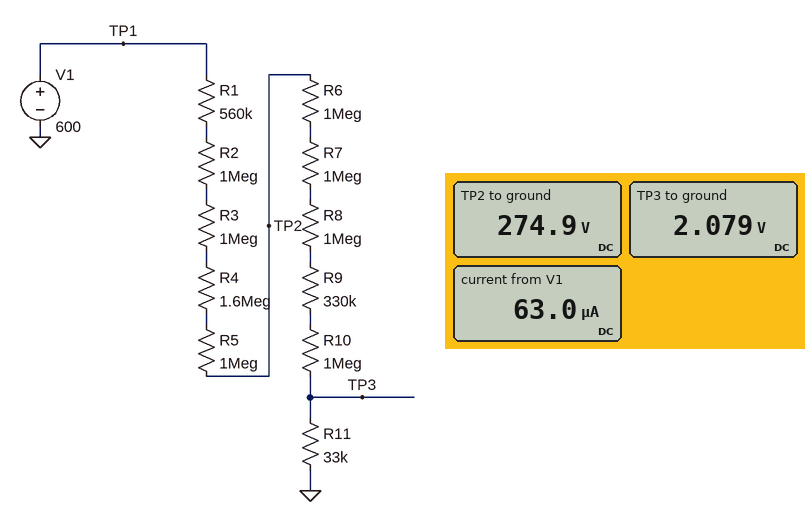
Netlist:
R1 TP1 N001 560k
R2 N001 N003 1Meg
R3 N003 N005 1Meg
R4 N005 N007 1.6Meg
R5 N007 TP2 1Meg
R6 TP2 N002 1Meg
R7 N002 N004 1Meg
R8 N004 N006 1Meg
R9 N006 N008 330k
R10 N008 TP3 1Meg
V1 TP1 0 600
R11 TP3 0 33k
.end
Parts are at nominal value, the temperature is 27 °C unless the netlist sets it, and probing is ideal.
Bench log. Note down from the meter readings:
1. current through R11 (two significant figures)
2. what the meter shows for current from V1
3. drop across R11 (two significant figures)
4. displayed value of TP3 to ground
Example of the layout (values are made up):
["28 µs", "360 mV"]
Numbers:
["63 µA", "63.0 µA", "2.1 V", "2.079 V"]
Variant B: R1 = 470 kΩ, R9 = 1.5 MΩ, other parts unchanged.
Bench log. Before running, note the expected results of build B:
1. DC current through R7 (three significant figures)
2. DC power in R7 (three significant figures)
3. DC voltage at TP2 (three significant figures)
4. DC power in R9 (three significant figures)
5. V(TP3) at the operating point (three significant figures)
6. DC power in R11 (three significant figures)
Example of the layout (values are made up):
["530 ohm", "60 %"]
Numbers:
["56.6 µA", "3.20 mW", "313 V", "4.80 mW", "1.87 V", "106 µW"]
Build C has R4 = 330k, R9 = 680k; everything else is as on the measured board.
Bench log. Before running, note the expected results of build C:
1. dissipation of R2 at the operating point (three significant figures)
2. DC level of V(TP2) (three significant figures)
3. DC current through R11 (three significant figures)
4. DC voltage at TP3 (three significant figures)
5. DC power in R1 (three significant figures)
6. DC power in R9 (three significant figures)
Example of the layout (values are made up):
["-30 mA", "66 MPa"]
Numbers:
["4.86 mW", "329 V", "69.7 µA", "2.30 V", "2.72 mW", "3.31 mW"]
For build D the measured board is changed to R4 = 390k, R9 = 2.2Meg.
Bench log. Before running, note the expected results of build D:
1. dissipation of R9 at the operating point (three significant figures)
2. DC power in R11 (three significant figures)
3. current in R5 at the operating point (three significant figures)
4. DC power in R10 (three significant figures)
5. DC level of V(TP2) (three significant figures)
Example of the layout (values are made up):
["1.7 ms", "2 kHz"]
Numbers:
["7.64 mW", "115 µW", "58.9 µA", "3.47 mW", "367 V"]
